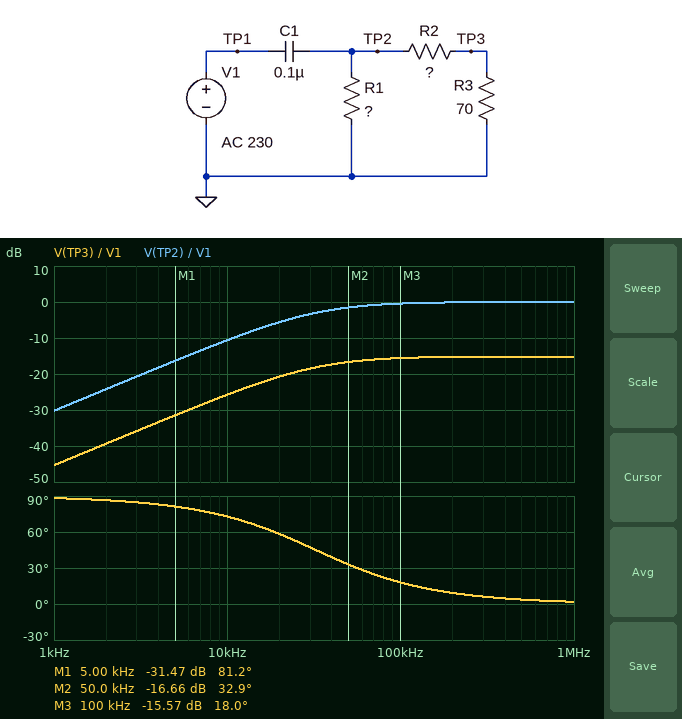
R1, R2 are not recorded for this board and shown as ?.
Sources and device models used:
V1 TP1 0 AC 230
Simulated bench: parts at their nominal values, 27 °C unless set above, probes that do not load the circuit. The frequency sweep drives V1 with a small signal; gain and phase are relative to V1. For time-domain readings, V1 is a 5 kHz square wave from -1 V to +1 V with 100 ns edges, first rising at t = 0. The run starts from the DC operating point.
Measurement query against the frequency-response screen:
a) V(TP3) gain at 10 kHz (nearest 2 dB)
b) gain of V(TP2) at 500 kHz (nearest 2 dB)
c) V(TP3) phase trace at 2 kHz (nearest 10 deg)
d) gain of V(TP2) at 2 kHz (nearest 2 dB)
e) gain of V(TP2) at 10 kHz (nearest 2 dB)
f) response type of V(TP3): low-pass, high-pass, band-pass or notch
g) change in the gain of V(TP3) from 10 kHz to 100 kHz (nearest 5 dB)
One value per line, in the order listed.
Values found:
-26 dB
0 dB
90 deg
-24 dB
-10 dB
high-pass
10 dB
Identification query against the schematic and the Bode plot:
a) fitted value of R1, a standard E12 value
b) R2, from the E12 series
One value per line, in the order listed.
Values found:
56 Ω
330 Ω
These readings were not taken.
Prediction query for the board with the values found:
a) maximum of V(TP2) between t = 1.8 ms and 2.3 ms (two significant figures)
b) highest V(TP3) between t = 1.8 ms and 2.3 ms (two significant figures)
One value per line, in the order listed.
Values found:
2.0 V
350 mV
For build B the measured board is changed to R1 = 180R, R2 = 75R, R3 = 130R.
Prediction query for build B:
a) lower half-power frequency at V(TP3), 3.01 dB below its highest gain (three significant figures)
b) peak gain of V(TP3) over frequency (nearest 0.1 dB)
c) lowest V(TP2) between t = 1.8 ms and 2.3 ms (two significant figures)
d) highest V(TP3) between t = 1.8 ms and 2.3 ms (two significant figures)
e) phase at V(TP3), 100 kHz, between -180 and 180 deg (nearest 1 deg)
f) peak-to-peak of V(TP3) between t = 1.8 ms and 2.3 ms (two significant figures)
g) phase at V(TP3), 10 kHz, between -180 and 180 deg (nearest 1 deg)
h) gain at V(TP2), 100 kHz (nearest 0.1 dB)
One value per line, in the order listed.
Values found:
16.6 kHz
-4.0 dB
-2.0 V
1.3 V
9 deg
2.5 V
59 deg
-0.1 dB
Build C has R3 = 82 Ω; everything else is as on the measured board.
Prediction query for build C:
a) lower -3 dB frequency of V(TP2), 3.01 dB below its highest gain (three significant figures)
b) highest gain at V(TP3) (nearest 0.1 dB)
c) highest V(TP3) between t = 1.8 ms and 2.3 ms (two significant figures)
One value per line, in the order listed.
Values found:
32.3 kHz
-14.0 dB
390 mV
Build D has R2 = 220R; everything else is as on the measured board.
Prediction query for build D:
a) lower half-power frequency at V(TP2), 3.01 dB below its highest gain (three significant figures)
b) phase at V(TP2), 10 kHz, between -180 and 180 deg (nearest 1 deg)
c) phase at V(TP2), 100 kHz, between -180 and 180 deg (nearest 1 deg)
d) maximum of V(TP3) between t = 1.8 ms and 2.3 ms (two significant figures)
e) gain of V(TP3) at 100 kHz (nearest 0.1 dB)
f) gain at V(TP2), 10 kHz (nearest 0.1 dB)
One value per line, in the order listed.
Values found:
33.9 kHz
74 deg
19 deg
480 mV
-12.8 dB
-11.0 dB
